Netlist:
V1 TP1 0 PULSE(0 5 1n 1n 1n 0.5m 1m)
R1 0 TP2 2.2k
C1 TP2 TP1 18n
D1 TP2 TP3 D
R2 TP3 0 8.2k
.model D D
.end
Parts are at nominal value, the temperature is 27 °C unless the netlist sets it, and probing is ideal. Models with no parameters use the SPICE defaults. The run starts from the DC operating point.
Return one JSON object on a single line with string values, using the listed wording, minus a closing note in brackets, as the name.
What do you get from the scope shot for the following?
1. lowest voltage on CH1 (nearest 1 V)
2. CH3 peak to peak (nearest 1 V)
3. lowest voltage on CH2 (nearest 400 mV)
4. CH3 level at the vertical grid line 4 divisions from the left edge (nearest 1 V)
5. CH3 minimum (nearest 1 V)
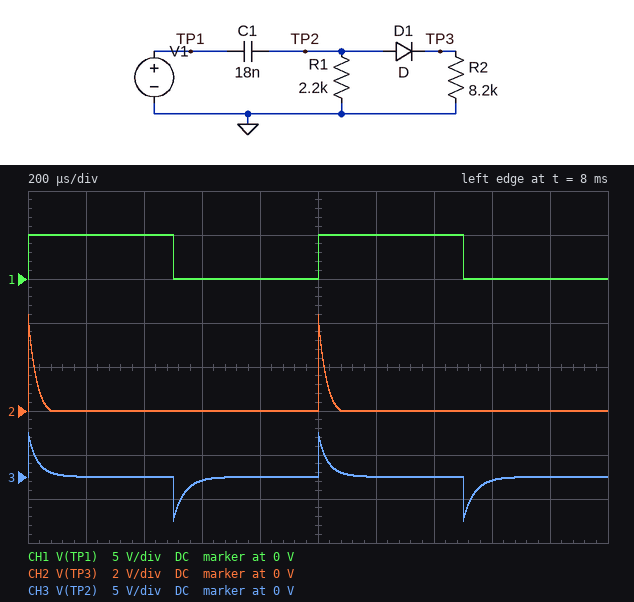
{"lowest voltage on CH1": "0 V", "CH3 peak to peak": "10 V", "lowest voltage on CH2": "0 V", "CH3 level at the vertical grid line 4 divisions from the left edge": "0 V", "CH3 minimum": "-5 V"}
